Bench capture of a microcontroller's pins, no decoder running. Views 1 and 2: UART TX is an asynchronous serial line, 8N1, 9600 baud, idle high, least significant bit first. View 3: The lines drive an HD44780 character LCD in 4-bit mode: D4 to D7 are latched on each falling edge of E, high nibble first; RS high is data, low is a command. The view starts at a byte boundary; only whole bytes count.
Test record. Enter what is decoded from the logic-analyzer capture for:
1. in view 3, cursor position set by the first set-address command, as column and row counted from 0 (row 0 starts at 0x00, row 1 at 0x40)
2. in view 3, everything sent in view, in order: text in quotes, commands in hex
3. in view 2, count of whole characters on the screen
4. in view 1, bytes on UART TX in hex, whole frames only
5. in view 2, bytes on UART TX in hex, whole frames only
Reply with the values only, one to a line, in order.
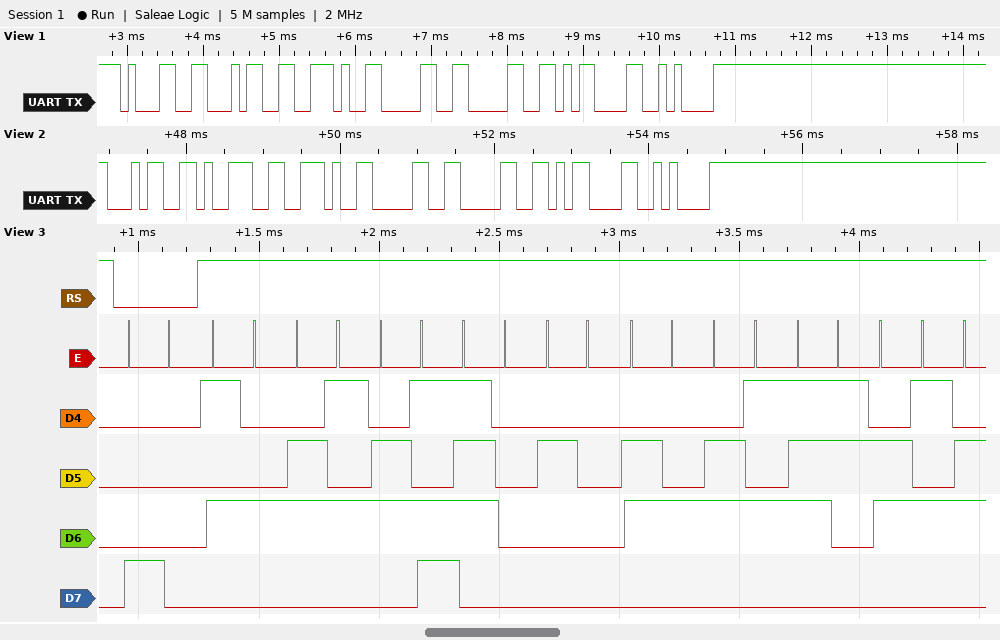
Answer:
column 0, row 0
0x80 "Temp dese"
7
0x31 0x34 0x2E 0x30 0x30 0x0D 0x0A
34 39 2E 30 30 0D 0A
